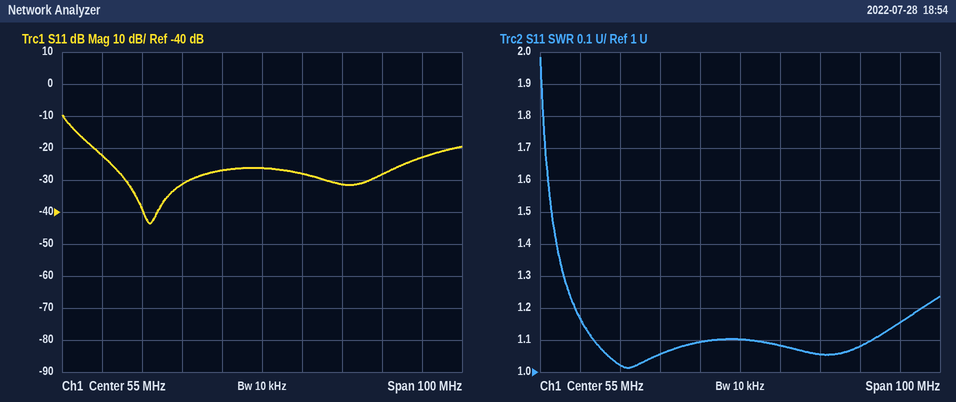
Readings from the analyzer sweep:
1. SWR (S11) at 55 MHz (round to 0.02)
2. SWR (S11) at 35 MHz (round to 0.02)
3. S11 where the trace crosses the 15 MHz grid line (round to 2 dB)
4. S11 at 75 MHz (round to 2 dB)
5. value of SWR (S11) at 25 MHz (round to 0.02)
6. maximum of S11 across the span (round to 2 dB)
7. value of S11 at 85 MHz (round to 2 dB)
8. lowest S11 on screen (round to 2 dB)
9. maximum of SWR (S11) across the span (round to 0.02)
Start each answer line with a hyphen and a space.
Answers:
- 1.10
- 1.06
- -22 dB
- -32 dB
- 1.02
- -10 dB
- -28 dB
- -44 dB
- 1.98
